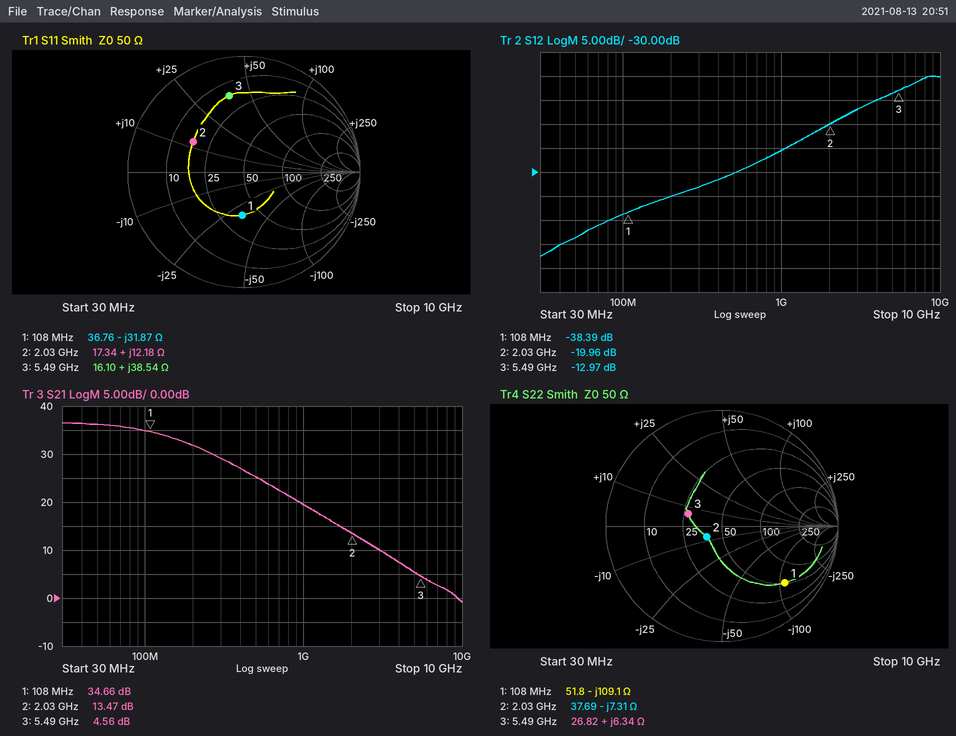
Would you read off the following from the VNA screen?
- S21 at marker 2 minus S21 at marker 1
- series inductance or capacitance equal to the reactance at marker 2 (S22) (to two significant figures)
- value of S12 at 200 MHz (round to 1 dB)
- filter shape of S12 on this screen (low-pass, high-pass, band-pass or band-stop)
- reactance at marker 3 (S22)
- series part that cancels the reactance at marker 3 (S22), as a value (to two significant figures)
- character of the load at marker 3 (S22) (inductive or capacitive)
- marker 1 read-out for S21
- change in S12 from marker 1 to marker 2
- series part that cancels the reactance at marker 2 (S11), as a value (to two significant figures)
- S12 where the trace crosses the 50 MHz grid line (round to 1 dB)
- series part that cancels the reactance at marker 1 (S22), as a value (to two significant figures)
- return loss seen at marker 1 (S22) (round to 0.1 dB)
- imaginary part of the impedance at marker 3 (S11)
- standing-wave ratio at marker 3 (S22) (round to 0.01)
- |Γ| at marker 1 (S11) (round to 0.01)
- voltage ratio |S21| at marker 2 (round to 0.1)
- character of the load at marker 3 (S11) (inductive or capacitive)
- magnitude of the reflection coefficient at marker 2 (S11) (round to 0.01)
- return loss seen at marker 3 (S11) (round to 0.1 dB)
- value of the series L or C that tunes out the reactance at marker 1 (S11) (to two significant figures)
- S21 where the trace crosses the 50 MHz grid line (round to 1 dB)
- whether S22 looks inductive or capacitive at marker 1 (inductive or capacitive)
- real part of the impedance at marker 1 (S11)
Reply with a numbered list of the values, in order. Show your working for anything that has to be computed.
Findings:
1. 13.47 − (34.66) = -21.19 dB
2. C = 1/(2π × 2.03 GHz × 7.31 Ω) ≈ 11 pF
3. -35 dB
4. high-pass
5. +6.34 Ω
6. C = 1/(2π × 5.49 GHz × 6.34 Ω) ≈ 4.6 pF
7. inductive
8. 34.66 dB
9. -19.96 − (-38.39) = 18.43 dB
10. C = 1/(2π × 2.03 GHz × 12.18 Ω) ≈ 6.4 pF
11. -44 dB
12. L = 109.1 Ω/(2π × 108 MHz) ≈ 161 nH, so 160 nH to two significant figures
13. 2.7 dB
14. +38.54 Ω
15. 1.91
16. 0.37
17. 10^(13.47/20) ≈ 4.7
18. inductive
19. 0.51
20. 3.5 dB
21. L = 31.87 Ω/(2π × 108 MHz) ≈ 47 nH
22. 36 dB
23. capacitive
24. 36.76 Ω
